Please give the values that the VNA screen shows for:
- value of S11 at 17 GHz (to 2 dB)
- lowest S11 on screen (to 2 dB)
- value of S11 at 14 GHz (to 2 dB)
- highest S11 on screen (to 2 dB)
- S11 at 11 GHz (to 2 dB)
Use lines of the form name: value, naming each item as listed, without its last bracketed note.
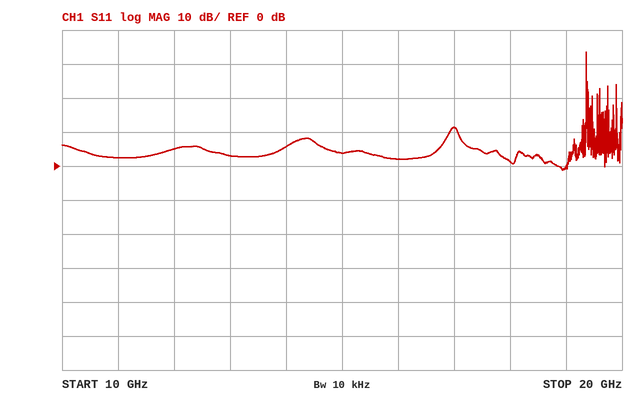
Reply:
value of S11 at 17 GHz: 12 dB
lowest S11 on screen: -2 dB
value of S11 at 14 GHz: 6 dB
highest S11 on screen: 34 dB
S11 at 11 GHz: 2 dB
